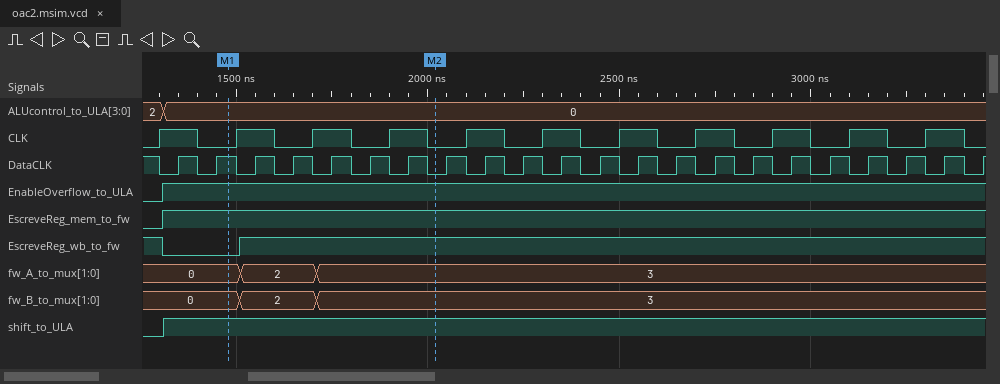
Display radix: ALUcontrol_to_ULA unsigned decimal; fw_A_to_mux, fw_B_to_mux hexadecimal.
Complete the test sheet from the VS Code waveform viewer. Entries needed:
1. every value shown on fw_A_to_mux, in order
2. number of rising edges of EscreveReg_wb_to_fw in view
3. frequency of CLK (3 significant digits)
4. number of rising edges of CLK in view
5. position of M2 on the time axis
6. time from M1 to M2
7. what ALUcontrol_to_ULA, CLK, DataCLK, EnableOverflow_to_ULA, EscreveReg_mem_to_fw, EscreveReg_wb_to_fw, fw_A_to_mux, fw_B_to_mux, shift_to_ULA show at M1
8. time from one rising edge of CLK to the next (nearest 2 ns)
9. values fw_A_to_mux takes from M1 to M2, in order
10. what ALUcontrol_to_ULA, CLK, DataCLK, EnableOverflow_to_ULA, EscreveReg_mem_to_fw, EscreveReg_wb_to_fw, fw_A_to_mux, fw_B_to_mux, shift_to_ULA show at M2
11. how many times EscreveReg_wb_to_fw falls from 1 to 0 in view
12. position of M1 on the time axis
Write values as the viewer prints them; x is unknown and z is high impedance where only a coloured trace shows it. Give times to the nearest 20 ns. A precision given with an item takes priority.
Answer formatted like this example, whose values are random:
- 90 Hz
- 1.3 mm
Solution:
- 0, 2, 3
- 1
- 5.00 MHz
- 11
- 2020 ns
- 540 ns
- ALUcontrol_to_ULA=0, CLK=0, DataCLK=1, EnableOverflow_to_ULA=1, EscreveReg_mem_to_fw=1, EscreveReg_wb_to_fw=0, fw_A_to_mux=0, fw_B_to_mux=0, shift_to_ULA=1
- 200 ns
- 0, 2, 3
- ALUcontrol_to_ULA=0, CLK=0, DataCLK=0, EnableOverflow_to_ULA=1, EscreveReg_mem_to_fw=1, EscreveReg_wb_to_fw=1, fw_A_to_mux=3, fw_B_to_mux=3, shift_to_ULA=1
- 1
- 1480 ns
